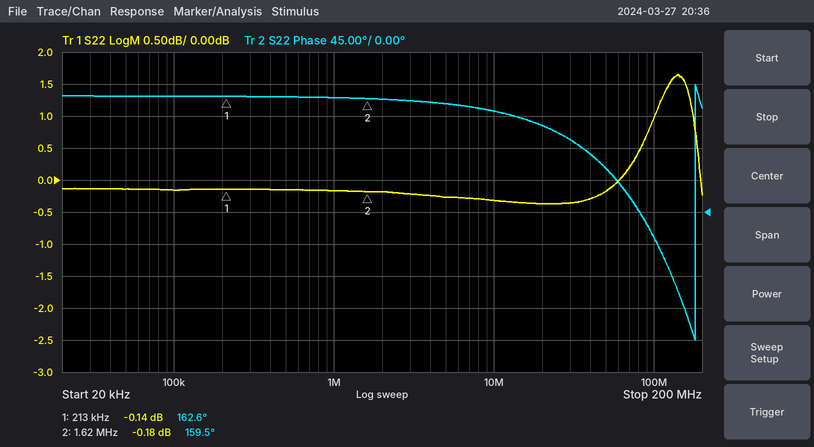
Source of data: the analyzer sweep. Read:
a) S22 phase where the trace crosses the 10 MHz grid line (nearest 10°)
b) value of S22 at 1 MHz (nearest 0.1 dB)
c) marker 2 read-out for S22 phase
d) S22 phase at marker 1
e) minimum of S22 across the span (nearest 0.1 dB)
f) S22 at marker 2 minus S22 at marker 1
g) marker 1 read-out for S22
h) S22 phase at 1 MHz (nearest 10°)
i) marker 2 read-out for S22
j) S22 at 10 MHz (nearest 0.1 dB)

140°
-0.2 dB
159.5°
162.6°
-0.4 dB
-0.04 dB
-0.14 dB
160°
-0.18 dB
-0.3 dB
